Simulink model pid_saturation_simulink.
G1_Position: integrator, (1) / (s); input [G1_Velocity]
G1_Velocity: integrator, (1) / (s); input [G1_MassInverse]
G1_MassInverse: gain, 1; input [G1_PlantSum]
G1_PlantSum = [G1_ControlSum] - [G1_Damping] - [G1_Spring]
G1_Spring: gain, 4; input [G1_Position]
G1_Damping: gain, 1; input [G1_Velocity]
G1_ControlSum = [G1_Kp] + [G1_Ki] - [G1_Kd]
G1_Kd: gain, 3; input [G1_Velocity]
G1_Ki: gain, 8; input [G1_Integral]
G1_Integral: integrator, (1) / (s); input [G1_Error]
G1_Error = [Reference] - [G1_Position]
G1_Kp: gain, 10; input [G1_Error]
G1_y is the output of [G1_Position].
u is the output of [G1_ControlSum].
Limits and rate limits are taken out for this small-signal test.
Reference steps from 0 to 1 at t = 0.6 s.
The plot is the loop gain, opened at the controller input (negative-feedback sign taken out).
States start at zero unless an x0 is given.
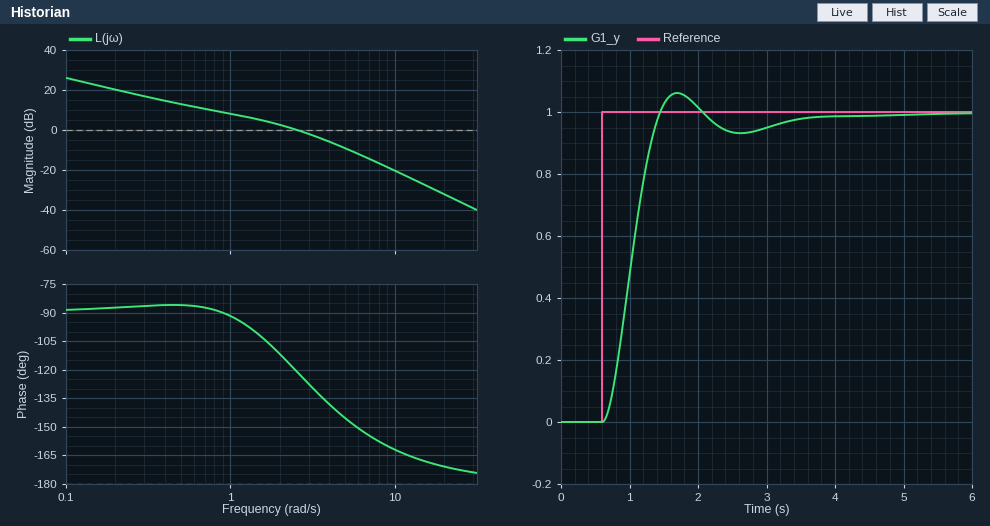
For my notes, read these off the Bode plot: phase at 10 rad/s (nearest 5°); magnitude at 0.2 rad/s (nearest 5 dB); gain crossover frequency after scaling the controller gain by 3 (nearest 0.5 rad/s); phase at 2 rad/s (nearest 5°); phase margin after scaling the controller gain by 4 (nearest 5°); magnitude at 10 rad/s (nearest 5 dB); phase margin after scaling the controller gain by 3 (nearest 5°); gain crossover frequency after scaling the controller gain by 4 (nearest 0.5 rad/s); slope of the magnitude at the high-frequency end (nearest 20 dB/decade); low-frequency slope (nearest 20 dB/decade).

-160°
20 dB
5.0 rad/s
-110°
30°
-20 dB
35°
6.0 rad/s
-40 dB/decade
-20 dB/decade
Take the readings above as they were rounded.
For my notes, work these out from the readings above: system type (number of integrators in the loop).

1
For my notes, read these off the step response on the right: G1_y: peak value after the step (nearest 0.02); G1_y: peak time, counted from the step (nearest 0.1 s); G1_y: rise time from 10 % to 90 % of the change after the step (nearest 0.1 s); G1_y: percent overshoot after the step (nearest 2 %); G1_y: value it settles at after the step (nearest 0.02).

1.06
1.1 s
0.6 s
6 %
1.00
